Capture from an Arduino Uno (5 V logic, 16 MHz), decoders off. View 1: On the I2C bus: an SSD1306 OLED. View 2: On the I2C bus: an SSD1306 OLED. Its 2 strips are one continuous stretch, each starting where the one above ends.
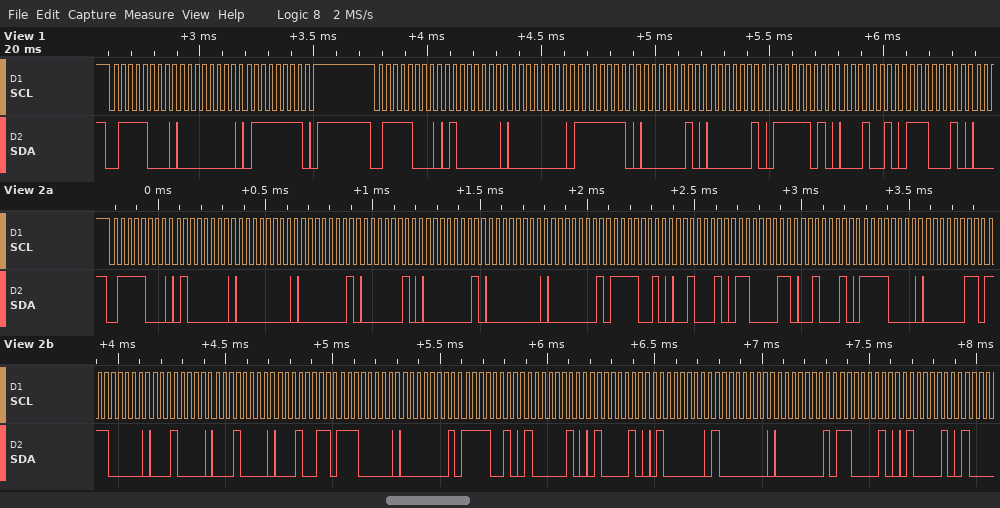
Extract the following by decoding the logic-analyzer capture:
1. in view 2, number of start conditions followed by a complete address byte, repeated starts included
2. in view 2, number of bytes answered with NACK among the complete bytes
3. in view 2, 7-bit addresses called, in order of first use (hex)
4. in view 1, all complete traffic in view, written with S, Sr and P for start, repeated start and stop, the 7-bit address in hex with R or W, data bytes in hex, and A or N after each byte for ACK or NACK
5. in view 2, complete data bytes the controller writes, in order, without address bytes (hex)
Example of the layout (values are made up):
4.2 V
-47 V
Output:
1
0
0x3C
S 3CW A 00 A 7F A P S 3CW A 40 A 00 A FE A 02 A 02 A FA A 12 A E2 A
40 00 01 02 01 00 01 F2 22 C3 22 F0 03 E0 10 10 13 E0 01 F2 82 42 40 80 01 C2 42
